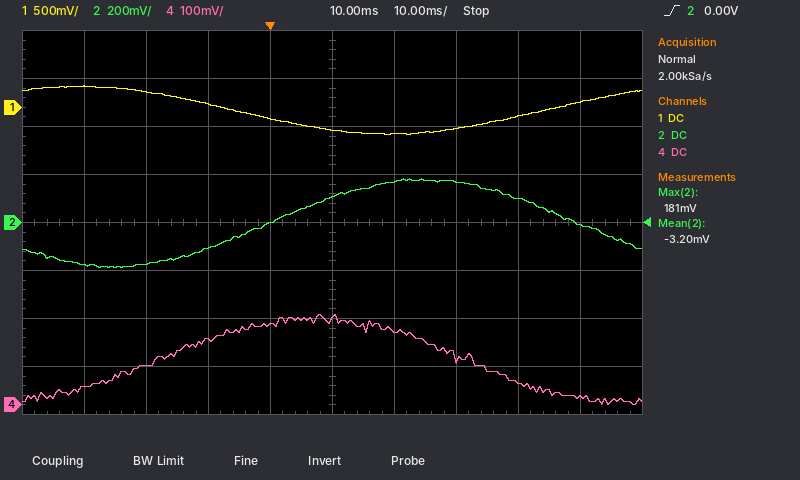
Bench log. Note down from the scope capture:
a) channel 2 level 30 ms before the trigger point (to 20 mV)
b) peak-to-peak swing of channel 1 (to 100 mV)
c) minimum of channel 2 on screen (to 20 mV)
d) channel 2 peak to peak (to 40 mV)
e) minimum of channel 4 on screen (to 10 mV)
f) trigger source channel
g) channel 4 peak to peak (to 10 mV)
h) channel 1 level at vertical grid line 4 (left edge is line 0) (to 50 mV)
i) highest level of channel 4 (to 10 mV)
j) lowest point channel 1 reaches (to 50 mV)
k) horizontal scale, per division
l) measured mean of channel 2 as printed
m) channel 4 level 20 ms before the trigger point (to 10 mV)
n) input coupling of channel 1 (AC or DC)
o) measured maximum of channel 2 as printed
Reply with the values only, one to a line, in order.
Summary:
-180 mV
500 mV
-180 mV
360 mV
0 mV
channel 2
190 mV
-100 mV
190 mV
-300 mV
10 ms
-3.20 mV
80 mV
DC
181 mV
